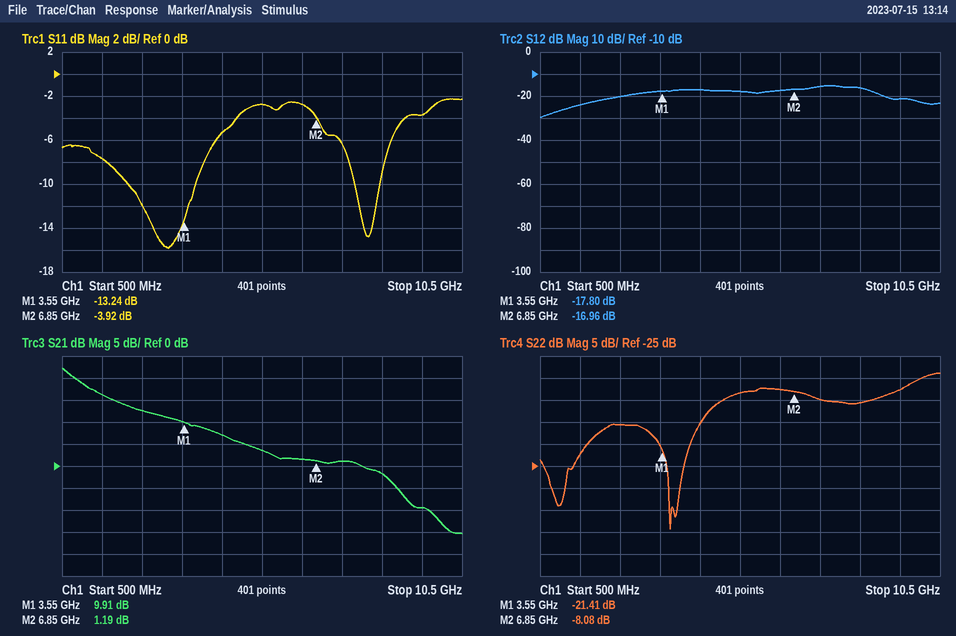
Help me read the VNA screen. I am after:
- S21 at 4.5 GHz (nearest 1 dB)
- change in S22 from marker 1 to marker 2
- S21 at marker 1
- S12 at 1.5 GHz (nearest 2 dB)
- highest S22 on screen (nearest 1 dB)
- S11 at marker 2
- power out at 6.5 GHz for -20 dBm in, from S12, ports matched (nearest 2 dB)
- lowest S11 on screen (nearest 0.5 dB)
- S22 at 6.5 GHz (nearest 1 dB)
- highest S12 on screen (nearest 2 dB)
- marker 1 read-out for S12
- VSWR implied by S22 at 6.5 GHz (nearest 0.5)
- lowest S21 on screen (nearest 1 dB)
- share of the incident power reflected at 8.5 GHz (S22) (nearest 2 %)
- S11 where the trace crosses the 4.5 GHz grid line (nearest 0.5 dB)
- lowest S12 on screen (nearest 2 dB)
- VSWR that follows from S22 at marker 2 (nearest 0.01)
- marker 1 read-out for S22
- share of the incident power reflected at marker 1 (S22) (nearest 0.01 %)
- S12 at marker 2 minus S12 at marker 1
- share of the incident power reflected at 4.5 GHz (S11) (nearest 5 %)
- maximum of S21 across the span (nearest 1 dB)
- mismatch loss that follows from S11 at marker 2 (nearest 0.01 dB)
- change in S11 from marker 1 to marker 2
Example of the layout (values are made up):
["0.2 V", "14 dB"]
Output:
["7 dB", "13.33 dB", "9.91 dB", "-24 dB", "-4 dB", "-3.92 dB", "-38 dBm", "-16.0 dB", "-8 dB", "-16 dB", "-17.80 dB", "2.5", "-15 dB", "8 %", "-5.5 dB", "-30 dB", "2.30", "-21.41 dB", "0.72 %", "0.84 dB", "30 %", "22 dB", "2.26 dB", "9.32 dB"]
